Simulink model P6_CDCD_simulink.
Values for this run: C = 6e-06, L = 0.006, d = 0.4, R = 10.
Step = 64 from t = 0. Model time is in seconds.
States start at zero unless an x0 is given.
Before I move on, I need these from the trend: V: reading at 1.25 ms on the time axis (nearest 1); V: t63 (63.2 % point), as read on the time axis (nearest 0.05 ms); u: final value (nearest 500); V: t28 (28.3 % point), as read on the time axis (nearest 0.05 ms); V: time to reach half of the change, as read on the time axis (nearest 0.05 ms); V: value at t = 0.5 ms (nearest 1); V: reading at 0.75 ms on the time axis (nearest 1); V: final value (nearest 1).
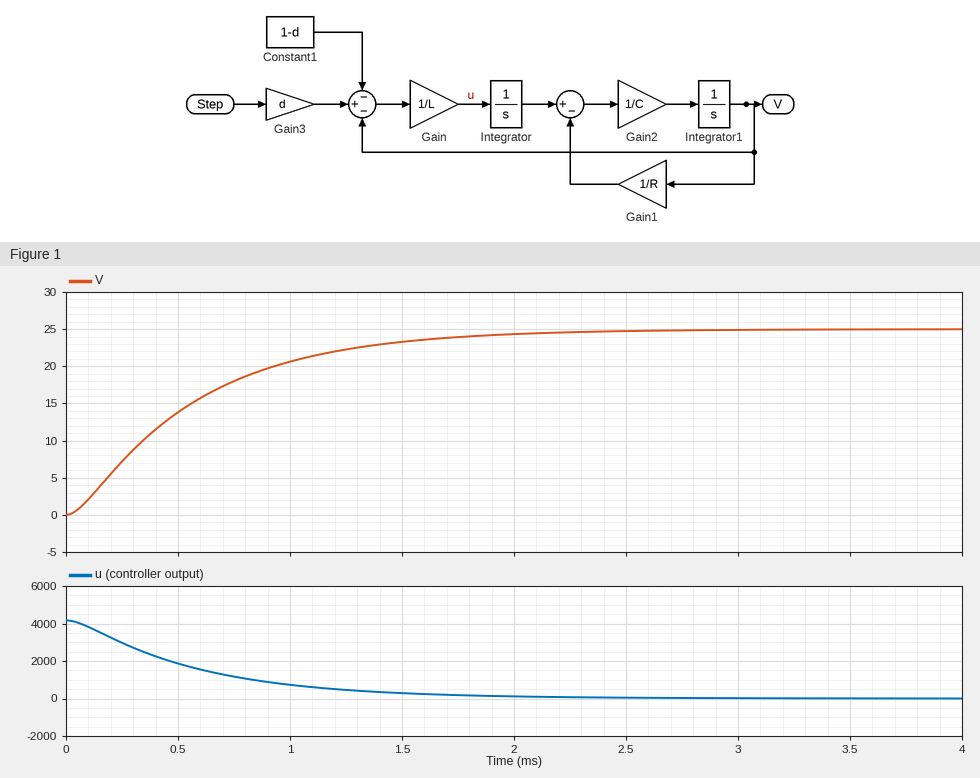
22
0.60 ms
0
0.25 ms
0.45 ms
14
18
25
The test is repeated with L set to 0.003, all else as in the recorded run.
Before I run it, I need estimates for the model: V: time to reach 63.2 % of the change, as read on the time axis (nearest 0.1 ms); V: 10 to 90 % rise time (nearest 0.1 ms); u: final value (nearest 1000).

0.3 ms
0.5 ms
0
